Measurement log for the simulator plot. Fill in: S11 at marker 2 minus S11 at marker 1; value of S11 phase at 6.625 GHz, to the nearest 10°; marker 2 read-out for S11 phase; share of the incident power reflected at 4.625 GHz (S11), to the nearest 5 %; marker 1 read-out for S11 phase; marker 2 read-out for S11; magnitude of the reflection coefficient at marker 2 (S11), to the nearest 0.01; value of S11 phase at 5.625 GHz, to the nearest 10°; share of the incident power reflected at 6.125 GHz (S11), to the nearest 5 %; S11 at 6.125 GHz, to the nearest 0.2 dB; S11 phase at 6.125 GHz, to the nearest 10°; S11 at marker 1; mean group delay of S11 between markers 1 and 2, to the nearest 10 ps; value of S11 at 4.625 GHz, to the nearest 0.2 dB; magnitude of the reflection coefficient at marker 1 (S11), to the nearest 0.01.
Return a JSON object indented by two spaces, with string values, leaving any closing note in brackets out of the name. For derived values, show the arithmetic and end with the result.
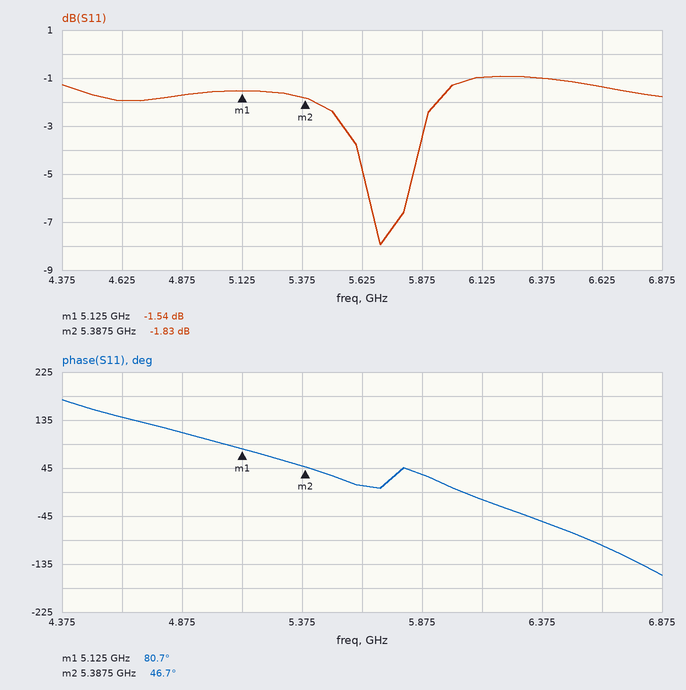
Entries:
{
  "S11 at marker 2 minus S11 at marker 1": "-1.83 − (-1.54) = -0.29 dB",
  "value of S11 phase at 6.625 GHz, to the nearest 10°": "-100°",
  "marker 2 read-out for S11 phase": "46.7°",
  "share of the incident power reflected at 4.625 GHz (S11), to the nearest 5 %": "10^(-2/10) ≈ 63.1 %, so 65 % to the nearest 5 %",
  "marker 1 read-out for S11 phase": "80.7°",
  "marker 2 read-out for S11": "-1.83 dB",
  "magnitude of the reflection coefficient at marker 2 (S11), to the nearest 0.01": "10^(-1.83/20) ≈ 0.81",
  "value of S11 phase at 5.625 GHz, to the nearest 10°": "10°",
  "share of the incident power reflected at 6.125 GHz (S11), to the nearest 5 %": "10^(-1/10) ≈ 79.4 %, so 80 % to the nearest 5 %",
  "S11 at 6.125 GHz, to the nearest 0.2 dB": "-1.0 dB",
  "S11 phase at 6.125 GHz, to the nearest 10°": "-10°",
  "S11 at marker 1": "-1.54 dB",
  "mean group delay of S11 between markers 1 and 2, to the nearest 10 ps": "−(46.7° − (80.7°))/(360° × 262.5 MHz) ≈ 360 ps",
  "value of S11 at 4.625 GHz, to the nearest 0.2 dB": "-2.0 dB",
  "magnitude of the reflection coefficient at marker 1 (S11), to the nearest 0.01": "10^(-1.54/20) ≈ 0.84"
}
